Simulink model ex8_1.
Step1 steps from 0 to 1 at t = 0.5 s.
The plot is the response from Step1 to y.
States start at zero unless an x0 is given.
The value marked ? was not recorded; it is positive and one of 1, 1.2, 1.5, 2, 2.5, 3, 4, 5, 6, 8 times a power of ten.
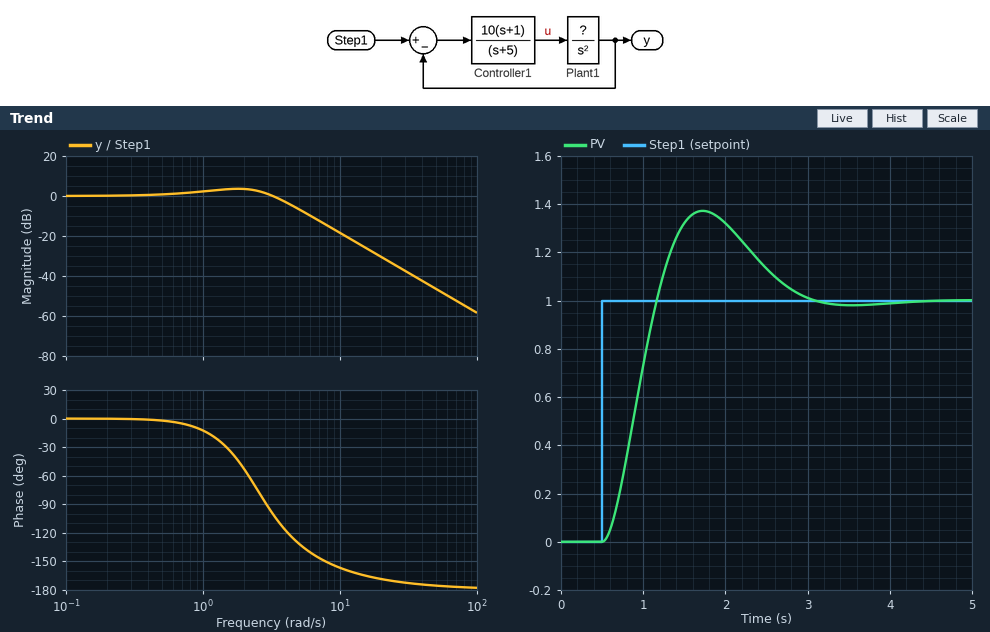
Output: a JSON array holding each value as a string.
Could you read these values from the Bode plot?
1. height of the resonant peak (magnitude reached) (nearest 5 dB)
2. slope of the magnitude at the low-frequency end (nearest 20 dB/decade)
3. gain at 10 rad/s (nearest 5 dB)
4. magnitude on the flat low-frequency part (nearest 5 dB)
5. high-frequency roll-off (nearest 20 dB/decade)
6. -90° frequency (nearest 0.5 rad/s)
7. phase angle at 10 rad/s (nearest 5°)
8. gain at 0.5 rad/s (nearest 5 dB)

["5 dB", "0 dB/decade", "-20 dB", "0 dB", "-40 dB/decade", "3.0 rad/s", "-155°", "0 dB"]
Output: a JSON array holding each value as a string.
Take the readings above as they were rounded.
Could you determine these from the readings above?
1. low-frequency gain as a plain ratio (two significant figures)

["1.0"]
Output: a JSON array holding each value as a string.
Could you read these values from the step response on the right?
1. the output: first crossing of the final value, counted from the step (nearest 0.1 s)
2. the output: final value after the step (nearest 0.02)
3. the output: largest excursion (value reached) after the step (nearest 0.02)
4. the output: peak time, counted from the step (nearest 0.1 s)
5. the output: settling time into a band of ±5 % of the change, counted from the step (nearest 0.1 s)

["0.7 s", "1.00", "1.38", "1.2 s", "2.3 s"]
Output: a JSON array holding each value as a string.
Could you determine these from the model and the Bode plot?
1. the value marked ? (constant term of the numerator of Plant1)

["1.2"]
